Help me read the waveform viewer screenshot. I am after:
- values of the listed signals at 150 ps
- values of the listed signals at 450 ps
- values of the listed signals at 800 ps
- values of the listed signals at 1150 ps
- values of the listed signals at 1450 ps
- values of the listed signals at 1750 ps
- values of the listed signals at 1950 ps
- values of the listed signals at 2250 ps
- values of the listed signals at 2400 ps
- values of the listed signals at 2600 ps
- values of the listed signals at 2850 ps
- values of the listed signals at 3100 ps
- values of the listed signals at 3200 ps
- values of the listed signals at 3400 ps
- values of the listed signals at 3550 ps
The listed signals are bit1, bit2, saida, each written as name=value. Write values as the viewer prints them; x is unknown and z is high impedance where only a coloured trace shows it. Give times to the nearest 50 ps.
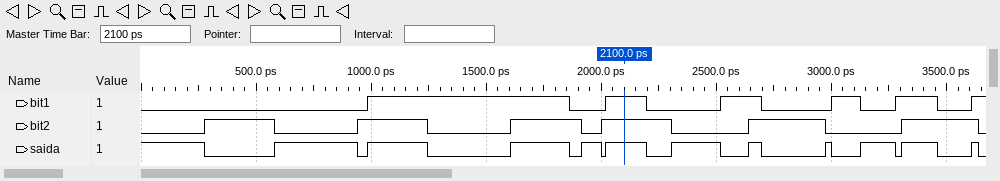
bit1=0, bit2=0, saida=1
bit1=0, bit2=1, saida=0
bit1=0, bit2=0, saida=1
bit1=1, bit2=1, saida=1
bit1=1, bit2=0, saida=0
bit1=1, bit2=1, saida=1
bit1=0, bit2=0, saida=1
bit1=0, bit2=1, saida=0
bit1=0, bit2=0, saida=1
bit1=1, bit2=0, saida=0
bit1=0, bit2=1, saida=0
bit1=1, bit2=0, saida=0
bit1=0, bit2=0, saida=1
bit1=1, bit2=1, saida=1
bit1=0, bit2=1, saida=0
